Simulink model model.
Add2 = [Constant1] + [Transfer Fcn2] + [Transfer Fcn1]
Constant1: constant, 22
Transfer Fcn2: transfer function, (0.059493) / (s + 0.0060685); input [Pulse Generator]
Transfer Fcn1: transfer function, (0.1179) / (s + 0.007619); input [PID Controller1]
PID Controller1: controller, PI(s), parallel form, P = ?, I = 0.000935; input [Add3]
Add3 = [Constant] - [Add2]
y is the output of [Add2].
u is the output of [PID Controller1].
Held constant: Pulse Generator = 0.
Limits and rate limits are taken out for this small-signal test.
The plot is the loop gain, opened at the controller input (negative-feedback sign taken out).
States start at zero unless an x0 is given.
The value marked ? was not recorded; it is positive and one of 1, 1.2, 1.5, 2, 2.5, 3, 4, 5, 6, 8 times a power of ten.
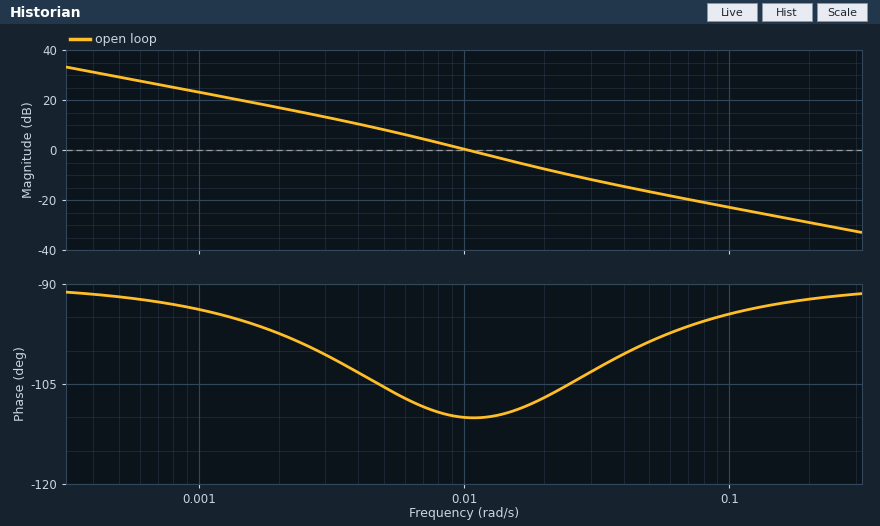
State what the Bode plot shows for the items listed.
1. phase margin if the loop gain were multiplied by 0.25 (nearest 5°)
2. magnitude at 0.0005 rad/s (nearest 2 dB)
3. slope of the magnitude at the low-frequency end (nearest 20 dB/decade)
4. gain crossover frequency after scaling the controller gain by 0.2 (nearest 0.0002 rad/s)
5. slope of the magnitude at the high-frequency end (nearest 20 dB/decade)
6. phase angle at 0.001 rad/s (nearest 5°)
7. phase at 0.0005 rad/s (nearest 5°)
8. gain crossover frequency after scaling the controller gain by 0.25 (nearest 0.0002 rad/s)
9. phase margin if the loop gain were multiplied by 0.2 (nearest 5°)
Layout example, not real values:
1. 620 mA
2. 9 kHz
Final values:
1. 80°
2. 30 dB
3. -20 dB/decade
4. 0.0028 rad/s
5. -20 dB/decade
6. -95°
7. -90°
8. 0.0034 rad/s
9. 80°
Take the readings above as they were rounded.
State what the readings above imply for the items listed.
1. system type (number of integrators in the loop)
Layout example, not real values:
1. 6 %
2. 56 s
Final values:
1. 1
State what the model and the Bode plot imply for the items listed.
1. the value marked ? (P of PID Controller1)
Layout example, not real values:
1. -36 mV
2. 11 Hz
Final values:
1. 0.06
